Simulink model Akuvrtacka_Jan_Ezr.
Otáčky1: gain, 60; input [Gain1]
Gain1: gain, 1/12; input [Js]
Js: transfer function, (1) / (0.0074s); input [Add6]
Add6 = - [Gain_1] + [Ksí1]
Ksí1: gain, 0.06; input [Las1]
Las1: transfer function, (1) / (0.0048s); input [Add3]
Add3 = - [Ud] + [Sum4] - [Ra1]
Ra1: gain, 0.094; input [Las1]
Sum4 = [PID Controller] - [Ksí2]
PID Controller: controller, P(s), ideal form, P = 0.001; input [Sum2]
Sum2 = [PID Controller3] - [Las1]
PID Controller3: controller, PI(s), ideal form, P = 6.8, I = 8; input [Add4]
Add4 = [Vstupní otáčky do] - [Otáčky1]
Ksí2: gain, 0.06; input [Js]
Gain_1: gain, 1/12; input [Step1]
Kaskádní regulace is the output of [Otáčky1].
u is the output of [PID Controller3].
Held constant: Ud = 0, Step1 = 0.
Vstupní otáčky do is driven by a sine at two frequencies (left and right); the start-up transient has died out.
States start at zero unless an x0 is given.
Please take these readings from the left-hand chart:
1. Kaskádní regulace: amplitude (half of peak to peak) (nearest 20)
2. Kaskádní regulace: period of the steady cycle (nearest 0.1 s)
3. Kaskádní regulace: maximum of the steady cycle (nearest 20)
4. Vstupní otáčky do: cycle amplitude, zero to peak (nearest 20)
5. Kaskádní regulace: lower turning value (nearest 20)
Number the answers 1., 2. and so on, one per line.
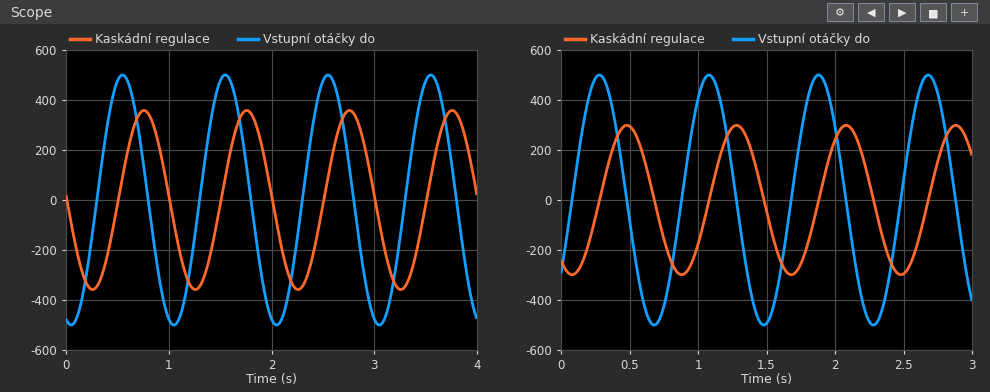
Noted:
1. 360
2. 1.0 s
3. 360
4. 500
5. -360
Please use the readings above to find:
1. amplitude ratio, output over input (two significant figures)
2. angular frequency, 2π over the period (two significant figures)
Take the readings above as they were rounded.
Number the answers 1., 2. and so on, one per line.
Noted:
1. 0.72
2. 6.3 rad/s
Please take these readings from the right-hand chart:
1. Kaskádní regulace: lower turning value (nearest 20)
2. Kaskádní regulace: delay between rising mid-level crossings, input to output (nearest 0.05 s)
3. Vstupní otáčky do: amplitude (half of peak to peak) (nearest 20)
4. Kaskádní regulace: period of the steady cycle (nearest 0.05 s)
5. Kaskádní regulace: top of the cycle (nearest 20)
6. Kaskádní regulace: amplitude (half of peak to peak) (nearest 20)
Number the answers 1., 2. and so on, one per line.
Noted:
1. -300
2. 0.20 s
3. 500
4. 0.80 s
5. 300
6. 300
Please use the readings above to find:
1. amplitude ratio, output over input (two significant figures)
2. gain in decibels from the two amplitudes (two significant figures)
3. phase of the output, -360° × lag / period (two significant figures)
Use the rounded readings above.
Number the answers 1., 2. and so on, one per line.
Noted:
1. 0.60
2. -4.4 dB
3. -90°
